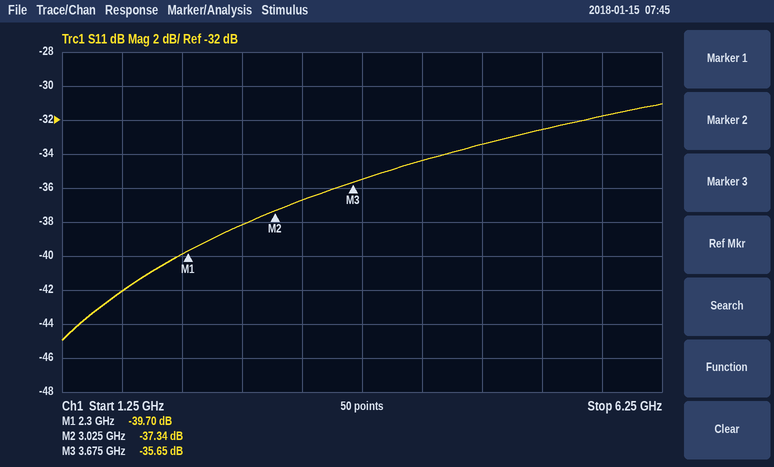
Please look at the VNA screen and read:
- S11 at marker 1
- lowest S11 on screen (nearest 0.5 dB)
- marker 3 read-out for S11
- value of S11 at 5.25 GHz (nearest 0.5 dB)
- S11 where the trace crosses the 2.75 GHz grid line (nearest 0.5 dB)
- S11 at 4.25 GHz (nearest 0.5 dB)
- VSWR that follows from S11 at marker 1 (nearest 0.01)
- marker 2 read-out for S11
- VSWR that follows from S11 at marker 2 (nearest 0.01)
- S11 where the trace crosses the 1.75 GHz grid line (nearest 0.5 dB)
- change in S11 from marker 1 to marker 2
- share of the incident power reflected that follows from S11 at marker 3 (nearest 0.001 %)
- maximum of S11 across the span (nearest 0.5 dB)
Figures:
-39.70 dB
-45.0 dB
-35.65 dB
-32.5 dB
-38.0 dB
-34.5 dB
1.02
-37.34 dB
1.03
-42.0 dB
2.36 dB
0.027 %
-31.0 dB
